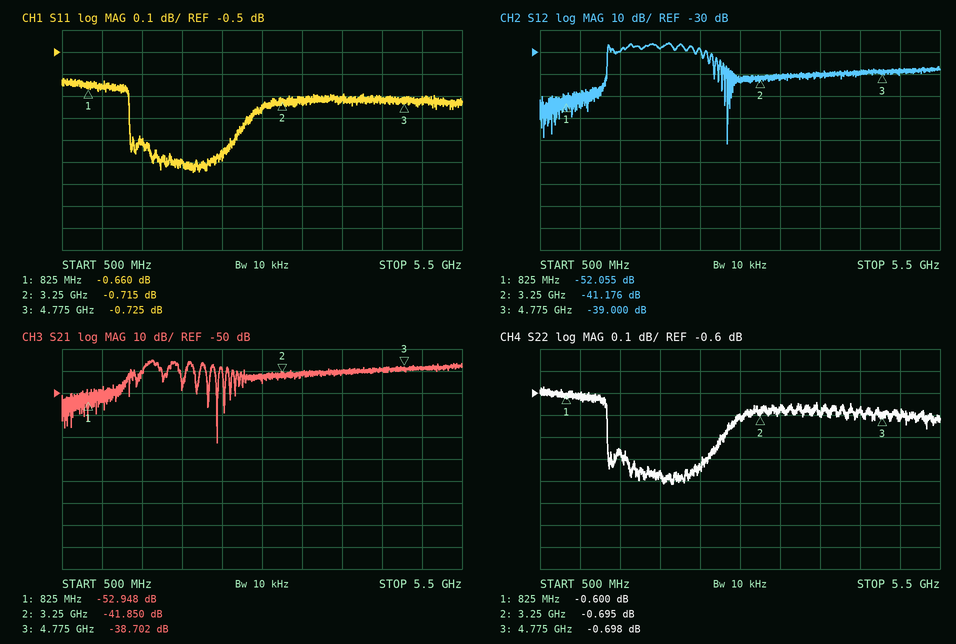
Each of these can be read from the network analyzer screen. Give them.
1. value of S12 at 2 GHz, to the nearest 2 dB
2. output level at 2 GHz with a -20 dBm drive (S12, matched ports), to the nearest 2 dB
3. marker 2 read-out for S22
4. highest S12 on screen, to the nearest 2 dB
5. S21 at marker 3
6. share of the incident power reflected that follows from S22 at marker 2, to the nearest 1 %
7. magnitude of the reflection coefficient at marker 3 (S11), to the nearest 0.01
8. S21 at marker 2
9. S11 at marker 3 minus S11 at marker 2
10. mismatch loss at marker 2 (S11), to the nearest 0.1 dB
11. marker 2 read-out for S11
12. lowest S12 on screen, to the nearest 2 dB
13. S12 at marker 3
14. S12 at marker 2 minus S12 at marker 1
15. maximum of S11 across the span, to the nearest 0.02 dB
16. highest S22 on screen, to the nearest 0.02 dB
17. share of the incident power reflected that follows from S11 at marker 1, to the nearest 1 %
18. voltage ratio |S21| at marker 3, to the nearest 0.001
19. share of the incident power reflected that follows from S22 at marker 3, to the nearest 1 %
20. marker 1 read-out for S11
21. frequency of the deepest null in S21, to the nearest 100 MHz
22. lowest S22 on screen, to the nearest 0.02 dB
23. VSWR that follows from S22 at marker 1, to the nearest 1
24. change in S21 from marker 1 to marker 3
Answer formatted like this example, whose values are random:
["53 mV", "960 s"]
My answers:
["-28 dB", "-48 dBm", "-0.695 dB", "-26 dB", "-38.702 dB", "85 %", "0.92", "-41.850 dB", "-0.010 dB", "8.2 dB", "-0.715 dB", "-72 dB", "-39.000 dB", "10.879 dB", "-0.62 dB", "-0.58 dB", "86 %", "0.012", "85 %", "-0.660 dB", "2.4 GHz", "-1.02 dB", "29", "14.246 dB"]
